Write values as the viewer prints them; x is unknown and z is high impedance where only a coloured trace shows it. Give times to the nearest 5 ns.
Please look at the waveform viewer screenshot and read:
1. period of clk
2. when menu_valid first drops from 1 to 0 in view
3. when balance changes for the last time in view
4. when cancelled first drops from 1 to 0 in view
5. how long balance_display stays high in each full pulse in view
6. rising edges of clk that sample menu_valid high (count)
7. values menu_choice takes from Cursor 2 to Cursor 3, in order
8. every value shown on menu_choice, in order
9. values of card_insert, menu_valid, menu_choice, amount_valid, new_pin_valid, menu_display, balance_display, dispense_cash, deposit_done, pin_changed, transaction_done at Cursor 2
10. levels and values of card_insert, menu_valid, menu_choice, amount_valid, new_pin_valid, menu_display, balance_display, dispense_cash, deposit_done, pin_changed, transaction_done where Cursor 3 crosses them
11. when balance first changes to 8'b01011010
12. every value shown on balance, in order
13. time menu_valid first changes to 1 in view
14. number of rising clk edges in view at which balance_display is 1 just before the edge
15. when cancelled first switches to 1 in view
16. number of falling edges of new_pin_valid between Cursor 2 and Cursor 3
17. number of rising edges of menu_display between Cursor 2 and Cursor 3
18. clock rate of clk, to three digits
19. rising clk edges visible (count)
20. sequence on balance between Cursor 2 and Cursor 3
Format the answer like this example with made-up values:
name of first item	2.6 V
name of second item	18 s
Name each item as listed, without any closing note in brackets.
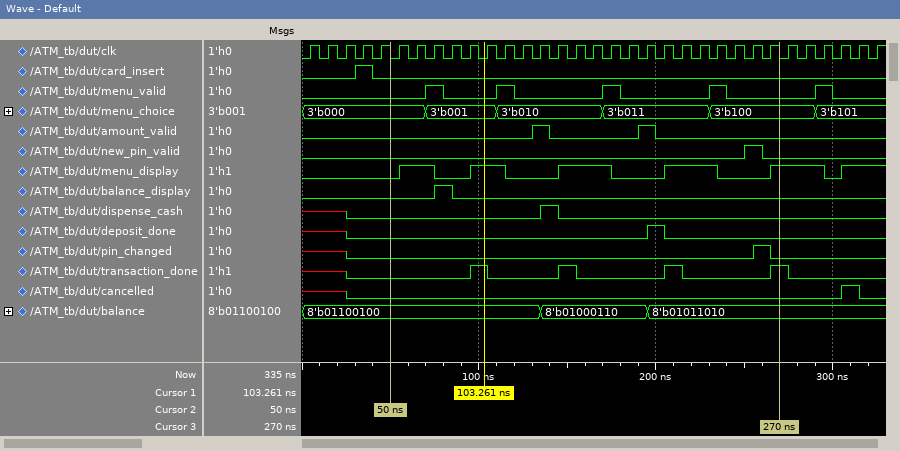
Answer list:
period of clk	10 ns
when menu_valid first drops from 1 to 0 in view	80 ns
when balance changes for the last time in view	195 ns
when cancelled first drops from 1 to 0 in view	315 ns
how long balance_display stays high in each full pulse in view	10 ns
rising edges of clk that sample menu_valid high	5
values menu_choice takes from Cursor 2 to Cursor 3, in order	3'b000, 3'b001, 3'b010, 3'b011, 3'b100
every value shown on menu_choice, in order	3'b000, 3'b001, 3'b010, 3'b011, 3'b100, 3'b101
values of card_insert, menu_valid, menu_choice, amount_valid, new_pin_valid, menu_display, balance_display, dispense_cash, deposit_done, pin_changed, transaction_done at Cursor 2	card_insert=0, menu_valid=0, menu_choice=3'b000, amount_valid=0, new_pin_valid=0, menu_display=0, balance_display=0, dispense_cash=0, deposit_done=0, pin_changed=0, transaction_done=0
levels and values of card_insert, menu_valid, menu_choice, amount_valid, new_pin_valid, menu_display, balance_display, dispense_cash, deposit_done, pin_changed, transaction_done where Cursor 3 crosses them	card_insert=0, menu_valid=0, menu_choice=3'b100, amount_valid=0, new_pin_valid=0, menu_display=1, balance_display=0, dispense_cash=0, deposit_done=0, pin_changed=0, transaction_done=1
when balance first changes to 8'b01011010	195 ns
every value shown on balance, in order	8'b01100100, 8'b01000110, 8'b01011010
time menu_valid first changes to 1 in view	70 ns
number of rising clk edges in view at which balance_display is 1 just before the edge	1
when cancelled first switches to 1 in view	305 ns
number of falling edges of new_pin_valid between Cursor 2 and Cursor 3	1
number of rising edges of menu_display between Cursor 2 and Cursor 3	5
clock rate of clk, to three digits	100 MHz
rising clk edges visible	33
sequence on balance between Cursor 2 and Cursor 3	8'b01100100, 8'b01000110, 8'b01011010
